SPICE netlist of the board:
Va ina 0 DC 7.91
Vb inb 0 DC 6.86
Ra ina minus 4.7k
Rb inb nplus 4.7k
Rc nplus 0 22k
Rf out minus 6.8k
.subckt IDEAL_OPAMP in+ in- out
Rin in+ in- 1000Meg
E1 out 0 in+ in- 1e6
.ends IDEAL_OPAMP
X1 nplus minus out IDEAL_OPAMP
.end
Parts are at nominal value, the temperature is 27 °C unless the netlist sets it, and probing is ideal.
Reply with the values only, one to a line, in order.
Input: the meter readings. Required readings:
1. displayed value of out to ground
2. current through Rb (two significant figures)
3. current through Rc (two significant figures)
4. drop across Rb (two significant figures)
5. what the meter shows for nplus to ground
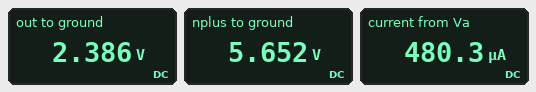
2.386 V
260 µA
260 µA
1.2 V
5.652 V
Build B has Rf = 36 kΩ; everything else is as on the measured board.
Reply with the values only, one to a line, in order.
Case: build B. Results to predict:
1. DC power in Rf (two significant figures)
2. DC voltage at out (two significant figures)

8.3 mW
-12 V
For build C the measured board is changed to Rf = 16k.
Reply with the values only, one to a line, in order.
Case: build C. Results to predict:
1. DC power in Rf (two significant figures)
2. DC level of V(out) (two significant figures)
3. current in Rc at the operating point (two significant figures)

3.7 mW
-2.0 V
260 µA
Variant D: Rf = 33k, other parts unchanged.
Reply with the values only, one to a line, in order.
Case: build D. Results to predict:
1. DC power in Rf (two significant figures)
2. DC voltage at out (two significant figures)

7.6 mW
-10 V
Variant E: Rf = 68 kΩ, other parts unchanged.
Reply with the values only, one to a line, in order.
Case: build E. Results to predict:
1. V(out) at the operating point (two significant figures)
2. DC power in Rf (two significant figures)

-27 V
16 mW
